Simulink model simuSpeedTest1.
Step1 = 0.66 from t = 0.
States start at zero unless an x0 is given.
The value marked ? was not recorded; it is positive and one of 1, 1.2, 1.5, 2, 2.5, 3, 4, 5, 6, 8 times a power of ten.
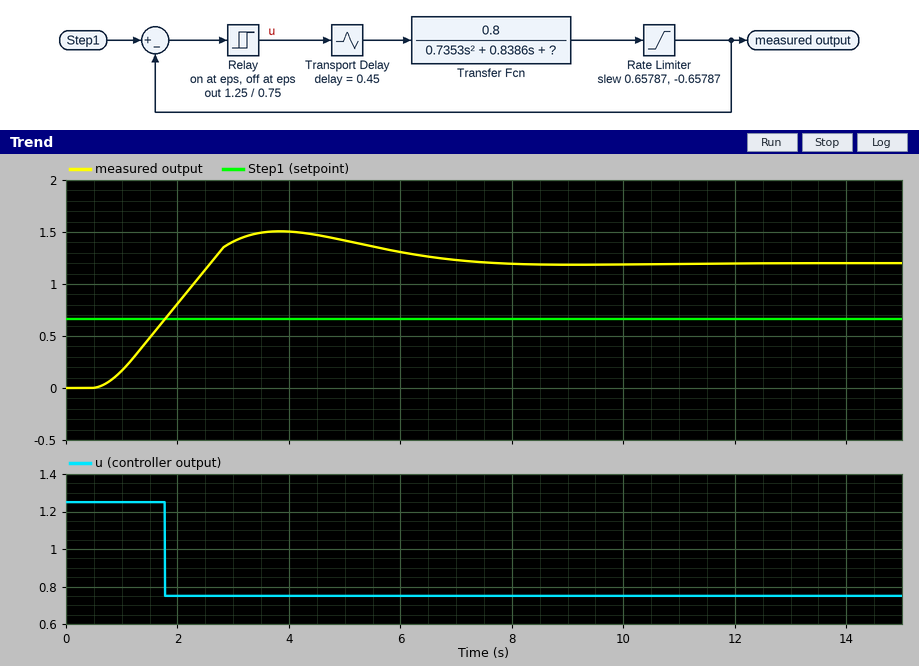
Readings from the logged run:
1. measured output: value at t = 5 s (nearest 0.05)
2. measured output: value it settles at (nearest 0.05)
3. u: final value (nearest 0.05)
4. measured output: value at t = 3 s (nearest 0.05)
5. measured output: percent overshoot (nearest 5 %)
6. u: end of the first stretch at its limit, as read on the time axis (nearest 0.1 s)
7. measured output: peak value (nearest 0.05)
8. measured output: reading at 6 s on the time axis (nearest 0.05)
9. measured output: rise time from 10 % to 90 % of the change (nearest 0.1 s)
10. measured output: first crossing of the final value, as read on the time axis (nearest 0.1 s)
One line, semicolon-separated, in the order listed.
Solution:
1.40; 1.20; 0.75; 1.40; 25 %; 1.8 s; 1.50; 1.30; 1.5 s; 2.6 s
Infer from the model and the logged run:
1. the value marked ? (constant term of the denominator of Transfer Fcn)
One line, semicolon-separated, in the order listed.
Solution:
0.5
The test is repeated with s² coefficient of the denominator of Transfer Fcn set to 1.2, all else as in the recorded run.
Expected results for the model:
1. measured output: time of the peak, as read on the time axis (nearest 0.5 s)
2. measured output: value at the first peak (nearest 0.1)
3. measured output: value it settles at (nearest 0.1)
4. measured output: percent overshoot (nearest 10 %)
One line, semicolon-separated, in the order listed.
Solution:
4.5 s; 1.6; 1.2; 40 %
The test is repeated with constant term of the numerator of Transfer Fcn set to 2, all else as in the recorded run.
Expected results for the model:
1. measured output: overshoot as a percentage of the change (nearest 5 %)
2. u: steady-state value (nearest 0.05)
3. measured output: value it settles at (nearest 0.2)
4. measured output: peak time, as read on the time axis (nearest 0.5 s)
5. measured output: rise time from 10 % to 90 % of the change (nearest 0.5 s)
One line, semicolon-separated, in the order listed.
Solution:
10 %; 0.75; 3.0; 5.5 s; 3.5 s
